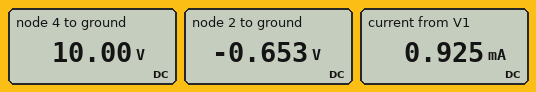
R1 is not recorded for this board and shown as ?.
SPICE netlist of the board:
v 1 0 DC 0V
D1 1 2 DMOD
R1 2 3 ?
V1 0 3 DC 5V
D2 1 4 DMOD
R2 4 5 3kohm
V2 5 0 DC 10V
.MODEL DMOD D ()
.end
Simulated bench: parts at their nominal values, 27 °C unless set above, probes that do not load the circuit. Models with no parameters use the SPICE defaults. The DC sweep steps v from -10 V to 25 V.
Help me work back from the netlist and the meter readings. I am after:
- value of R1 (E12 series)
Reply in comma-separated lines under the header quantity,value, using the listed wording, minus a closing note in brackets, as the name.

quantity,value
value of R1,4.7 kΩ
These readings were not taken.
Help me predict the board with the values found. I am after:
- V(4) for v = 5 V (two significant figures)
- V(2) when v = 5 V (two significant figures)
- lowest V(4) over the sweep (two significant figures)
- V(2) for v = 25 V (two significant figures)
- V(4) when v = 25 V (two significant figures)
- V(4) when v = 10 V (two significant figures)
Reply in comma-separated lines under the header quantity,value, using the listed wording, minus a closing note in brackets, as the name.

quantity,value
V(4) for v = 5 V,10 V
V(2) when v = 5 V,4.3 V
lowest V(4) over the sweep,10 V
V(2) for v = 25 V,24 V
V(4) when v = 25 V,24 V
V(4) when v = 10 V,10 V
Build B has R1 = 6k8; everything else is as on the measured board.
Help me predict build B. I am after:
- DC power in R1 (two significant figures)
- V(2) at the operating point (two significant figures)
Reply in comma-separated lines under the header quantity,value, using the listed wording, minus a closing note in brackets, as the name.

quantity,value
DC power in R1,2.8 mW
V(2) at the operating point,-640 mV
